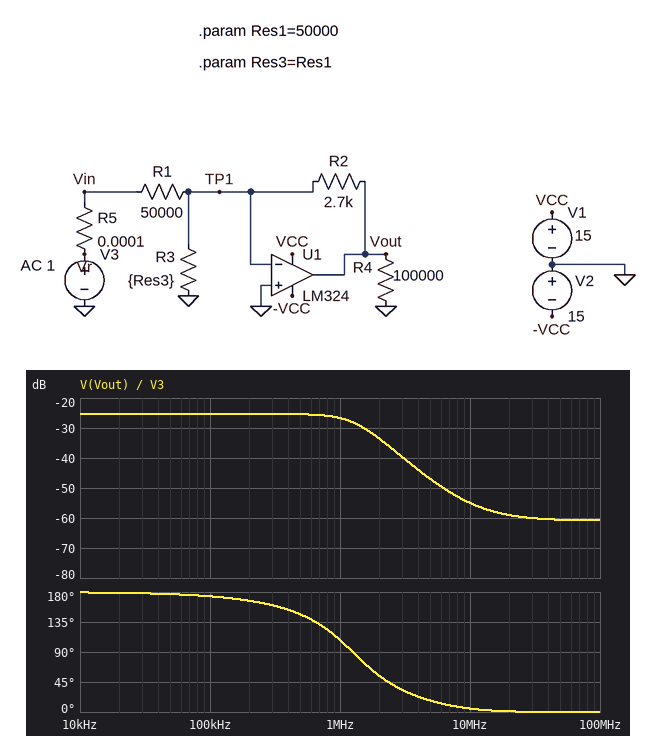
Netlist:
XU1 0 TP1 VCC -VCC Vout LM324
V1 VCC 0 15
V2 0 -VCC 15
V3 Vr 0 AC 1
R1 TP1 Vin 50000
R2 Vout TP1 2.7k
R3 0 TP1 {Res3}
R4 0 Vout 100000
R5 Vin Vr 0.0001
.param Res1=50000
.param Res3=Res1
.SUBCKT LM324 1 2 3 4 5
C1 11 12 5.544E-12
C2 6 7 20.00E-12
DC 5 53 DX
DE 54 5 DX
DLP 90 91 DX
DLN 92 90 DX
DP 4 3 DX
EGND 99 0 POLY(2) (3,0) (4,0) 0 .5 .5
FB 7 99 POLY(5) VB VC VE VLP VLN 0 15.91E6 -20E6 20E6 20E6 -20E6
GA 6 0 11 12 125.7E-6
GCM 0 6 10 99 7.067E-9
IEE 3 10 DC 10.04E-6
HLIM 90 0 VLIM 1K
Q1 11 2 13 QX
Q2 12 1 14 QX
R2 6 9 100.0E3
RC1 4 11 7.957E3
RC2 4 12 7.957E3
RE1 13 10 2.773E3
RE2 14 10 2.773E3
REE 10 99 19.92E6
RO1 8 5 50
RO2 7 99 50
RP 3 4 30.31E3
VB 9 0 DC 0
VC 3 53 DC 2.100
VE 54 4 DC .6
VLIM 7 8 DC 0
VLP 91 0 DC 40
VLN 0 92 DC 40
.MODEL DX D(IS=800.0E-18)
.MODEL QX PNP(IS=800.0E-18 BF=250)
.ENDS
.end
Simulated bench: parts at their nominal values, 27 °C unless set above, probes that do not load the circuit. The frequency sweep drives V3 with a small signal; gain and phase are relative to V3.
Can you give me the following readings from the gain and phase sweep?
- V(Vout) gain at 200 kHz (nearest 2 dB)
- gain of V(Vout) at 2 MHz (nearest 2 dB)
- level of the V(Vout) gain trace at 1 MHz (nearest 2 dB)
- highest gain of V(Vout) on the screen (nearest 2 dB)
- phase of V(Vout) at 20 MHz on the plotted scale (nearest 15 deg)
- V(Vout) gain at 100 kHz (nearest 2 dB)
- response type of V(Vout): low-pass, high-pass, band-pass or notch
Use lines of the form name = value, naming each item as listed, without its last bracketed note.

V(Vout) gain at 200 kHz = -26 dB
gain of V(Vout) at 2 MHz = -34 dB
level of the V(Vout) gain trace at 1 MHz = -26 dB
highest gain of V(Vout) on the screen = -26 dB
phase of V(Vout) at 20 MHz on the plotted scale = 0 deg
V(Vout) gain at 100 kHz = -26 dB
response type of V(Vout): low-pass, high-pass, band-pass or notch = low-pass
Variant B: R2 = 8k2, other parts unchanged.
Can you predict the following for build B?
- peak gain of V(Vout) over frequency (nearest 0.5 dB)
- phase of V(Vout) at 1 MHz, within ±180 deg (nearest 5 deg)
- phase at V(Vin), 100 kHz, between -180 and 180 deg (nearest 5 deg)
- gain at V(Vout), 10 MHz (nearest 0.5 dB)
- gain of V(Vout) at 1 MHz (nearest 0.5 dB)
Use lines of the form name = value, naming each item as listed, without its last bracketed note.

peak gain of V(Vout) over frequency = -15.5 dB
phase of V(Vout) at 1 MHz, within ±180 deg = 100 deg
phase at V(Vin), 100 kHz, between -180 and 180 deg = 0 deg
gain at V(Vout), 10 MHz = -50.5 dB
gain of V(Vout) at 1 MHz = -18.5 dB
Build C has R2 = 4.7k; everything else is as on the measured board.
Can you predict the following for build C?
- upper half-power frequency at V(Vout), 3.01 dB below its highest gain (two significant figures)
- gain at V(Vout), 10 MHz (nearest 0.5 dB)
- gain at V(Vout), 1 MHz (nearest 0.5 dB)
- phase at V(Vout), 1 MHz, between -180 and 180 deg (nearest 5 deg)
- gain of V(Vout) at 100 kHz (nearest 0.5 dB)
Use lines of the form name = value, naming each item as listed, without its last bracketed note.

upper half-power frequency at V(Vout), 3.01 dB below its highest gain = 1.2 MHz
gain at V(Vout), 10 MHz = -53.0 dB
gain at V(Vout), 1 MHz = -22.5 dB
phase at V(Vout), 1 MHz, between -180 and 180 deg = 105 deg
gain of V(Vout) at 100 kHz = -20.5 dB
